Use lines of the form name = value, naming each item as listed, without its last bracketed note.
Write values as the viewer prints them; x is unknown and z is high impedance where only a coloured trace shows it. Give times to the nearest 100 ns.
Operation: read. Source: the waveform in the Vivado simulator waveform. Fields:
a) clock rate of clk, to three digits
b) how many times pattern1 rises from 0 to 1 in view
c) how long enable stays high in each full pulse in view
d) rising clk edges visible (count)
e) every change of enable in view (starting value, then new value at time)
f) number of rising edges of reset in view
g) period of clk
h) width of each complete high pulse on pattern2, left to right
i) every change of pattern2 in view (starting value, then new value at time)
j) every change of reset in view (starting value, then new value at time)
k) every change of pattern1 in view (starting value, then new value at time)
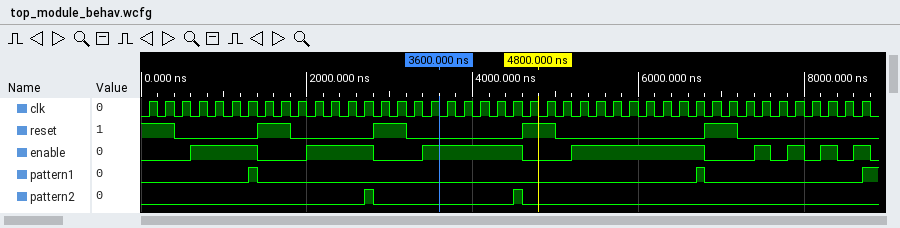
clock rate of clk, to three digits = 5.00 MHz
how many times pattern1 rises from 0 to 1 in view = 3
how long enable stays high in each full pulse in view = 800 ns, 800 ns, 1200 ns, 1600 ns, 200 ns, 200 ns, 200 ns, 200 ns
rising clk edges visible = 44
every change of enable in view = 0, 1 at 600 ns, 0 at 1400 ns, 1 at 2000 ns, 0 at 2800 ns, 1 at 3400 ns, 0 at 4600 ns, 1 at 5200 ns, 0 at 6800 ns, 1 at 7400 ns, 0 at 7600 ns, 1 at 7800 ns, 0 at 8000 ns, 1 at 8200 ns, 0 at 8400 ns, 1 at 8600 ns, 0 at 8800 ns
number of rising edges of reset in view = 4
period of clk = 200 ns
width of each complete high pulse on pattern2, left to right = 100 ns, 100 ns
every change of pattern2 in view = 0, 1 at 2700 ns, 0 at 2800 ns, 1 at 4500 ns, 0 at 4600 ns
every change of reset in view = 1, 0 at 400 ns, 1 at 1400 ns, 0 at 1800 ns, 1 at 2800 ns, 0 at 3200 ns, 1 at 4600 ns, 0 at 5000 ns, 1 at 6800 ns, 0 at 7200 ns
every change of pattern1 in view = 0, 1 at 1300 ns, 0 at 1400 ns, 1 at 6700 ns, 0 at 6800 ns, 1 at 8700 ns
